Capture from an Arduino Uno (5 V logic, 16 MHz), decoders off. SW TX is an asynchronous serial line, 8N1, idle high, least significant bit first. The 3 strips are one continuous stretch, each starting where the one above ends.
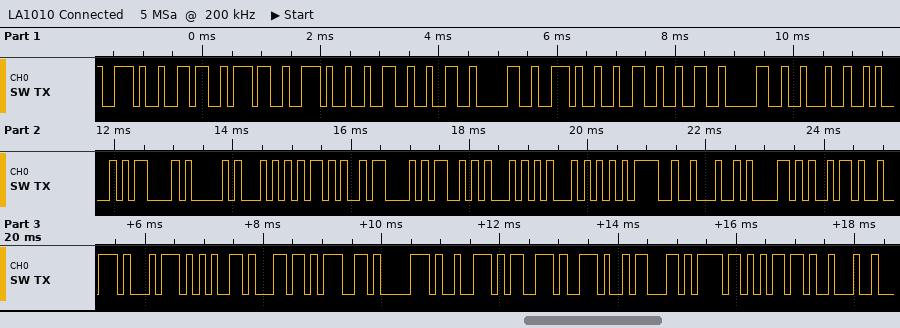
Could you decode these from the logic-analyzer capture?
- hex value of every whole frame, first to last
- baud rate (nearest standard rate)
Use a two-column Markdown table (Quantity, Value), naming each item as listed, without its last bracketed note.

| Quantity | Value |
|---|---|
| hex value of every whole frame, first to last | 2E 36 37 2E 32 32 30 2E 32 32 30 22 0A 0D 41 54 2B 43 53 54 54 3D 22 61 69 72 74 65 6C 67 70 72 73 2E 63 6F 6D 22 |
| baud rate | 9600 baud |
